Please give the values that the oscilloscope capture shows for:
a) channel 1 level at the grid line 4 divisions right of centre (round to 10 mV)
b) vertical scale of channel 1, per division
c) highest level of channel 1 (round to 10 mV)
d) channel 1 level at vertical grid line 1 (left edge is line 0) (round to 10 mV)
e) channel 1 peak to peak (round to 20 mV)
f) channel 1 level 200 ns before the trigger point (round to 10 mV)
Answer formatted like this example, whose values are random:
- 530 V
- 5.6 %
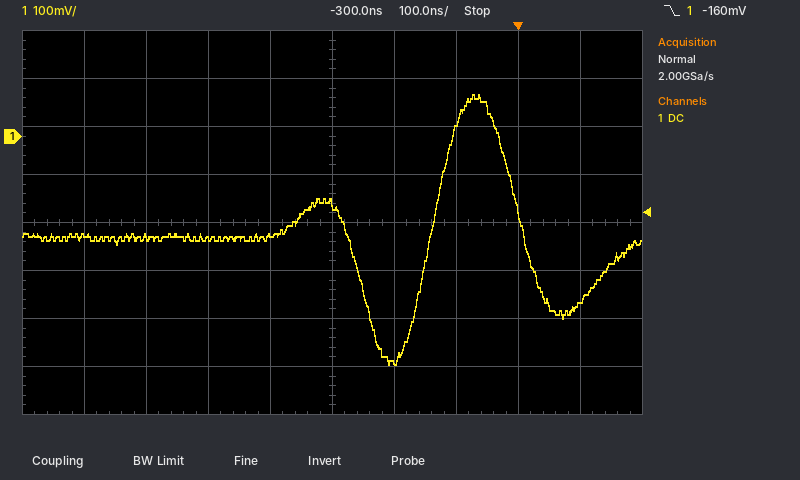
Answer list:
- -350 mV
- 100 mV
- 90 mV
- -210 mV
- 560 mV
- -470 mV
